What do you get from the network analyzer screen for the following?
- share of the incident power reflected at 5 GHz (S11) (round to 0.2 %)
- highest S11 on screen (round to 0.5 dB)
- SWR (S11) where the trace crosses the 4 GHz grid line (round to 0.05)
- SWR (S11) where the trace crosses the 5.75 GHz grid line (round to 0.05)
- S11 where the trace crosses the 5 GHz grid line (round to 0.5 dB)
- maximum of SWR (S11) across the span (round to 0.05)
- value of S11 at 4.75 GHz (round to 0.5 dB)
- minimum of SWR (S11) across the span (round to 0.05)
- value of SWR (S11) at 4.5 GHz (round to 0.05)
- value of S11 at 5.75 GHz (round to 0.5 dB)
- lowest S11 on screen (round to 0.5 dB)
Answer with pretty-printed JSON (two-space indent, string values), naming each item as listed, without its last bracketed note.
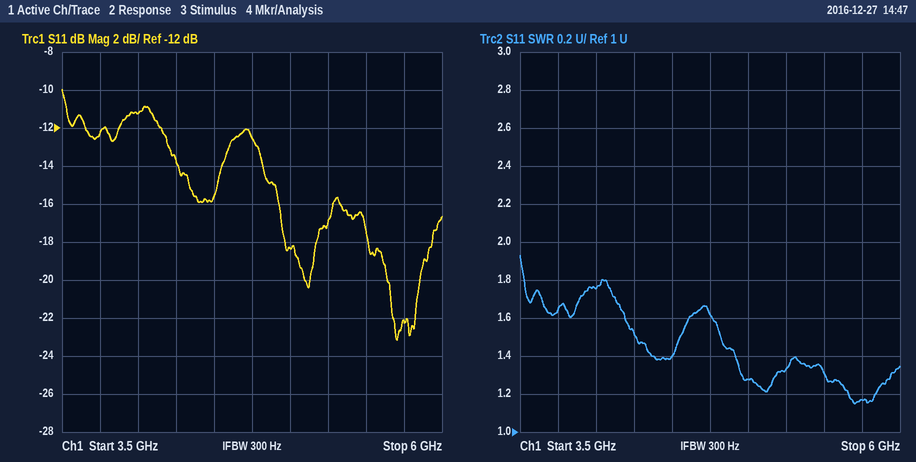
{
  "share of the incident power reflected at 5 GHz (S11)": "1.4 %",
  "highest S11 on screen": "-10.0 dB",
  "SWR (S11) where the trace crosses the 4 GHz grid line": "1.75",
  "SWR (S11) where the trace crosses the 5.75 GHz grid line": "1.15",
  "S11 where the trace crosses the 5 GHz grid line": "-18.5 dB",
  "maximum of SWR (S11) across the span": "1.95",
  "value of S11 at 4.75 GHz": "-12.5 dB",
  "minimum of SWR (S11) across the span": "1.15",
  "value of SWR (S11) at 4.5 GHz": "1.40",
  "value of S11 at 5.75 GHz": "-22.0 dB",
  "lowest S11 on screen": "-23.0 dB"
}
